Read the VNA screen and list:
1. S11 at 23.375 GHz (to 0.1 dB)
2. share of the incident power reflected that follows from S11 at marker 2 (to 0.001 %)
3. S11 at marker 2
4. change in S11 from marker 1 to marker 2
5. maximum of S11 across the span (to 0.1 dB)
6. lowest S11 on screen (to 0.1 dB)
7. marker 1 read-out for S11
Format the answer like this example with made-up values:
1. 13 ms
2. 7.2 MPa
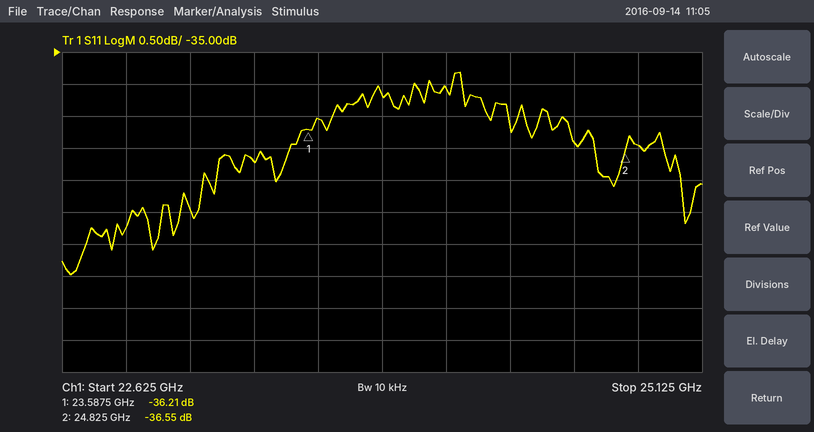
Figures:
1. -36.7 dB
2. 0.022 %
3. -36.55 dB
4. -0.34 dB
5. -35.3 dB
6. -38.5 dB
7. -36.21 dB
